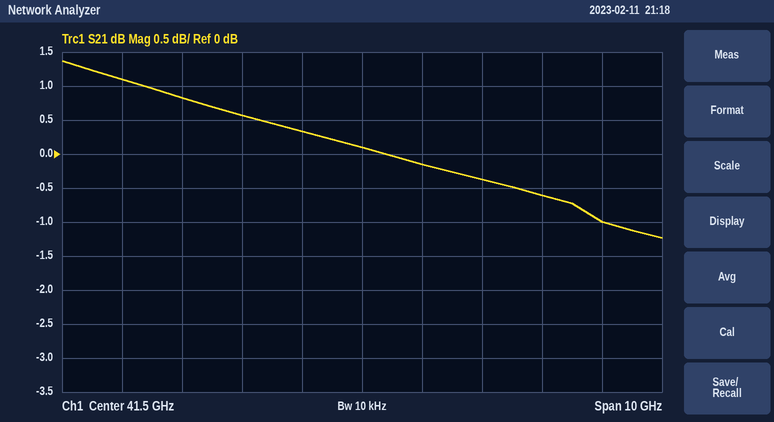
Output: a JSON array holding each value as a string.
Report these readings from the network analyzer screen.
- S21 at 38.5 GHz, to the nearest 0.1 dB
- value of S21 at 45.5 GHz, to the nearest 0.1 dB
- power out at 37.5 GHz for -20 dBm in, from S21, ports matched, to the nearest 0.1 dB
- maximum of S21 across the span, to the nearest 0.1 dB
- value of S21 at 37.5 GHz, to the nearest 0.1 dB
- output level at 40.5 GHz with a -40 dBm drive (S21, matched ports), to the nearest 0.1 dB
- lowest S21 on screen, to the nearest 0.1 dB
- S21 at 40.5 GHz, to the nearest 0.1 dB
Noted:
["0.8 dB", "-1.0 dB", "-18.9 dBm", "1.4 dB", "1.1 dB", "-39.7 dBm", "-1.2 dB", "0.3 dB"]
